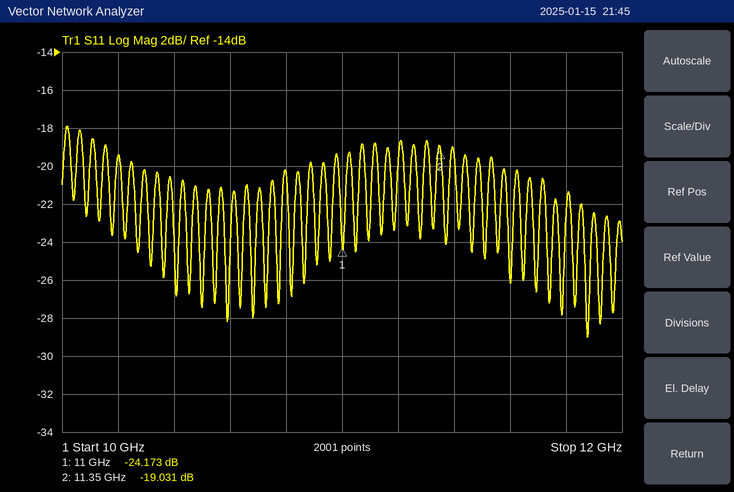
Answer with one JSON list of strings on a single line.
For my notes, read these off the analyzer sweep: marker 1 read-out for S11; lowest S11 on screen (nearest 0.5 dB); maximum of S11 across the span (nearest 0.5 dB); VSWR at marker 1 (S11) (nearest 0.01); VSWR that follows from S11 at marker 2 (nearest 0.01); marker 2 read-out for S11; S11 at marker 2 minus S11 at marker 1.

["-24.173 dB", "-29.0 dB", "-18.0 dB", "1.13", "1.25", "-19.031 dB", "5.142 dB"]
